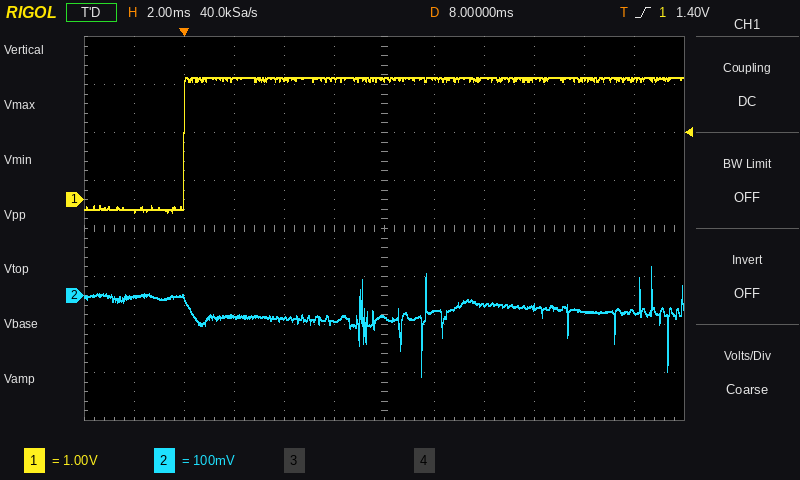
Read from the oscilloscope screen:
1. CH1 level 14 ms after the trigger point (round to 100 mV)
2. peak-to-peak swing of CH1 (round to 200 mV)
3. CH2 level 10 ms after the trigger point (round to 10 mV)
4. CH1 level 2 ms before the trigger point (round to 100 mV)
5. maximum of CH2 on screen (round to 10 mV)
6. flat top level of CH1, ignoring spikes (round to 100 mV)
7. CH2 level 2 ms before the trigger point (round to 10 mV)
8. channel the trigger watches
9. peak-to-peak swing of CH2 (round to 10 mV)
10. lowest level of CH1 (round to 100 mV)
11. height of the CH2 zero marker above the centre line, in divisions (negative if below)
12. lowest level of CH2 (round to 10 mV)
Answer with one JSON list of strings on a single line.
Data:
["2.5 V", "2.8 V", "-30 mV", "-200 mV", "60 mV", "2.5 V", "0 mV", "CH1", "230 mV", "-300 mV", "-1.4 div", "-170 mV"]
